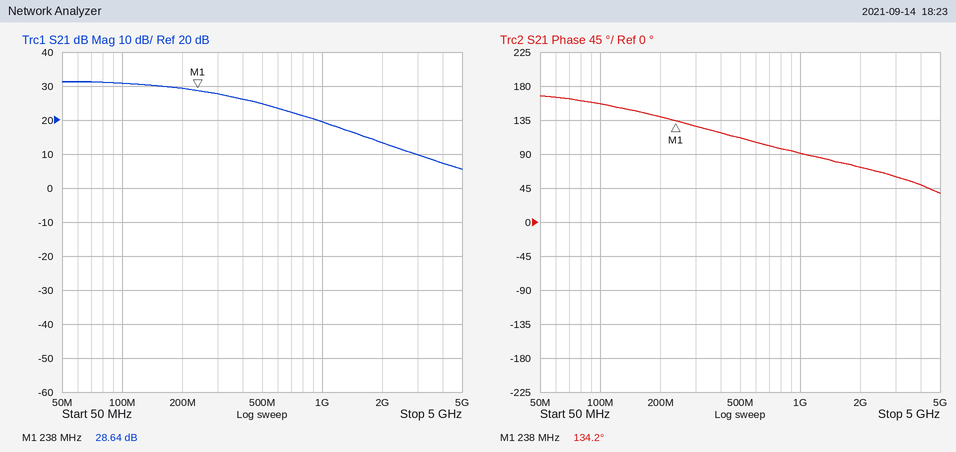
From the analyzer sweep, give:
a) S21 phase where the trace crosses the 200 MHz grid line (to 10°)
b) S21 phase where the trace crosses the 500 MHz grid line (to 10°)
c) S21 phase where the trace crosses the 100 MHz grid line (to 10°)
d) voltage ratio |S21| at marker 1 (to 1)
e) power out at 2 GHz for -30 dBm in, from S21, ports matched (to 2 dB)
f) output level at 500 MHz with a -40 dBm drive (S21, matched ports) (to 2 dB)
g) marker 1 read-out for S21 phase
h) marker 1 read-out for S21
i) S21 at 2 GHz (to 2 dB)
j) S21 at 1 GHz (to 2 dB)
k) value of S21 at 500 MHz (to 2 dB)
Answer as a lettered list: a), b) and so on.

a) 140°
b) 110°
c) 160°
d) 27
e) -16 dBm
f) -16 dBm
g) 134.2°
h) 28.64 dB
i) 14 dB
j) 20 dB
k) 24 dB
